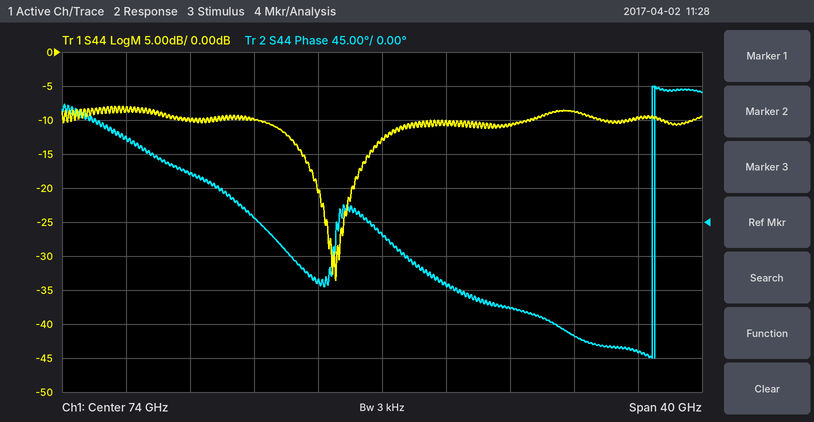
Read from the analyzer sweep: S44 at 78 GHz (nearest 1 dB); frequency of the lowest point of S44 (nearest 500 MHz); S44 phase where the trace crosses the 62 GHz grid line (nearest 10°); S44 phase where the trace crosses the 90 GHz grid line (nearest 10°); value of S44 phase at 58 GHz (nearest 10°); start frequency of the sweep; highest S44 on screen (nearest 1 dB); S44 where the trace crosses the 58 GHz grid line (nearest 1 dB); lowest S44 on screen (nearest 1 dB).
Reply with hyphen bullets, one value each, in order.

- -10 dB
- 71.0 GHz
- 60°
- -170°
- 110°
- 54 GHz
- -8 dB
- -8 dB
- -34 dB
